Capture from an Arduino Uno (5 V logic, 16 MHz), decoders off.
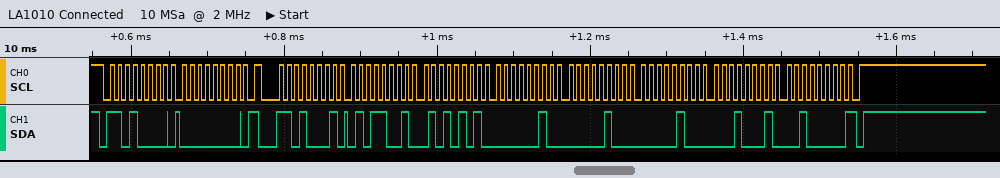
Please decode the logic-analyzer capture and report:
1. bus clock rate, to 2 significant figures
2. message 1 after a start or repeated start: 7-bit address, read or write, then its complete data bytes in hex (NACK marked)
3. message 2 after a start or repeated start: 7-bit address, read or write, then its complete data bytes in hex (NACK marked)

100 kHz
0x68 write: 00
0x68 read: 59 55 02 04 04 11 20 NACK
